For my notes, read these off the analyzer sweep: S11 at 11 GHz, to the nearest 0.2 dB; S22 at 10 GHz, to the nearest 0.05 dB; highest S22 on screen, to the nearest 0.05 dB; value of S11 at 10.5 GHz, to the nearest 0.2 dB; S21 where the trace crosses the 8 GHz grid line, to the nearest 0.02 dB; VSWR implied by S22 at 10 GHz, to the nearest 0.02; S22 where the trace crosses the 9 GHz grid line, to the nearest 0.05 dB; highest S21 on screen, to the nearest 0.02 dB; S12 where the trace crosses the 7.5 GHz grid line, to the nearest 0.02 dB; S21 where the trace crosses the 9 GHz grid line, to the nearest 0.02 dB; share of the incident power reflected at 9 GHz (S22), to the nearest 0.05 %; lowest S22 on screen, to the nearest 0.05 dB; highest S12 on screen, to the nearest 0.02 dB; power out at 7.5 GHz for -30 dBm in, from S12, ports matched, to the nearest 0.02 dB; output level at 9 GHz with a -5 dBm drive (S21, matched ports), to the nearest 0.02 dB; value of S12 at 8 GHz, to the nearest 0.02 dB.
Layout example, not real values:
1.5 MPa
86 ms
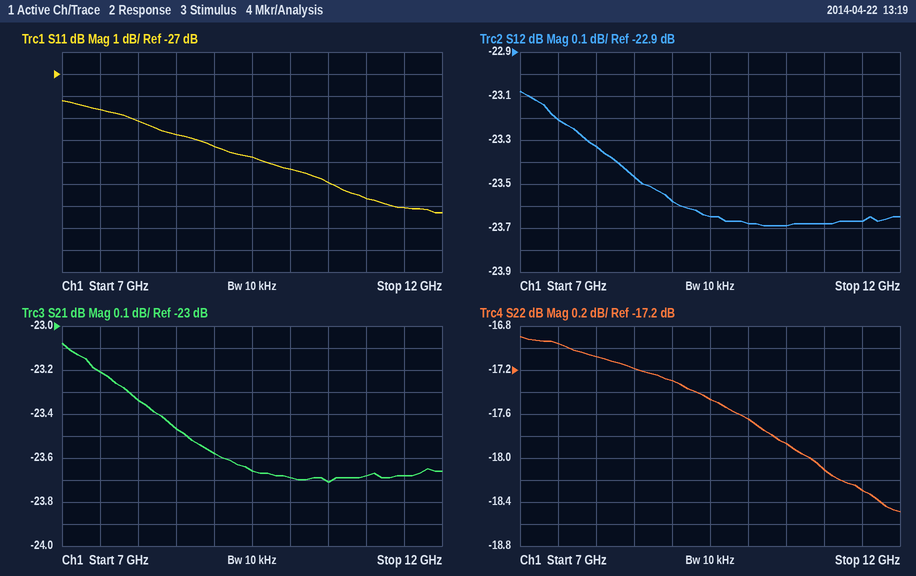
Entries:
-32.6 dB
-17.65 dB
-16.90 dB
-32.0 dB
-23.34 dB
1.30
-17.30 dB
-23.08 dB
-23.20 dB
-23.58 dB
1.85 %
-18.50 dB
-23.08 dB
-53.20 dBm
-28.58 dBm
-23.32 dB
